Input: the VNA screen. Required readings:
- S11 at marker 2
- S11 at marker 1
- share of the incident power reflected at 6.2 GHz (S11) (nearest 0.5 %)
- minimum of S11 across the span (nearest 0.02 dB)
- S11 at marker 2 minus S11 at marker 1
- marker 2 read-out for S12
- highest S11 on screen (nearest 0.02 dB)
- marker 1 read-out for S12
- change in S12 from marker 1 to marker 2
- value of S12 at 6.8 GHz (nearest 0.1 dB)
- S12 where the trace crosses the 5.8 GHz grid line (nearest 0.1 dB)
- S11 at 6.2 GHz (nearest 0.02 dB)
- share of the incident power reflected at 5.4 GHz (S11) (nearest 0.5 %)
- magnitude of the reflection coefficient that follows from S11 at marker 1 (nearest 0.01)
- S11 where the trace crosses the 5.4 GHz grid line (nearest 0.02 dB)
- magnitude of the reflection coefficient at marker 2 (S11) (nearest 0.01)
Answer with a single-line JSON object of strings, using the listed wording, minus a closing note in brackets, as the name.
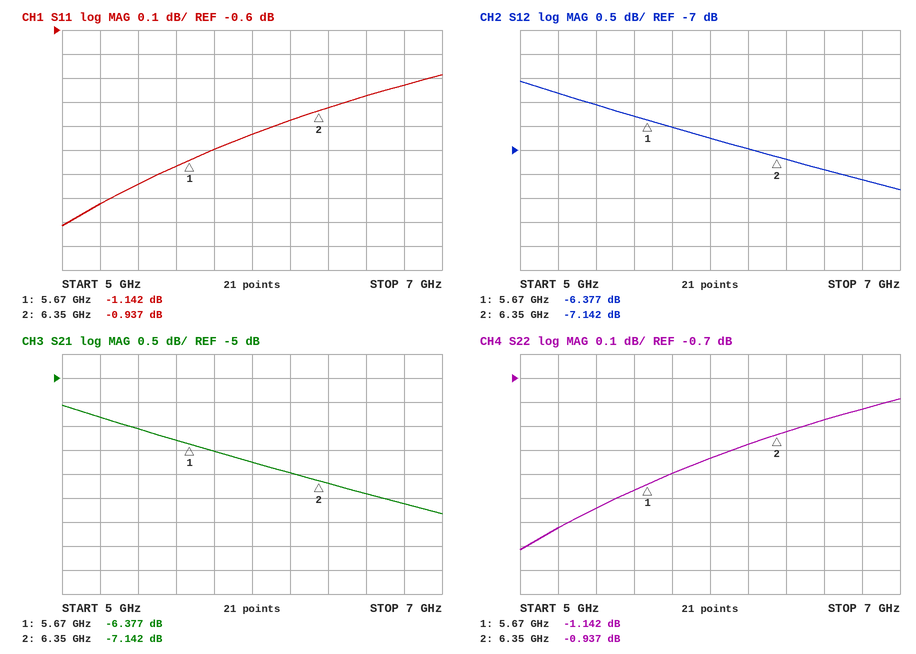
{"S11 at marker 2": "-0.937 dB", "S11 at marker 1": "-1.142 dB", "share of the incident power reflected at 6.2 GHz (S11)": "80.0 %", "minimum of S11 across the span": "-1.42 dB", "S11 at marker 2 minus S11 at marker 1": "0.205 dB", "marker 2 read-out for S12": "-7.142 dB", "highest S11 on screen": "-0.78 dB", "marker 1 read-out for S12": "-6.377 dB", "change in S12 from marker 1 to marker 2": "-0.765 dB", "value of S12 at 6.8 GHz": "-7.6 dB", "S12 where the trace crosses the 5.8 GHz grid line": "-6.5 dB", "S11 at 6.2 GHz": "-0.98 dB", "share of the incident power reflected at 5.4 GHz (S11)": "75.0 %", "magnitude of the reflection coefficient that follows from S11 at marker 1": "0.88", "S11 where the trace crosses the 5.4 GHz grid line": "-1.24 dB", "magnitude of the reflection coefficient at marker 2 (S11)": "0.90"}
